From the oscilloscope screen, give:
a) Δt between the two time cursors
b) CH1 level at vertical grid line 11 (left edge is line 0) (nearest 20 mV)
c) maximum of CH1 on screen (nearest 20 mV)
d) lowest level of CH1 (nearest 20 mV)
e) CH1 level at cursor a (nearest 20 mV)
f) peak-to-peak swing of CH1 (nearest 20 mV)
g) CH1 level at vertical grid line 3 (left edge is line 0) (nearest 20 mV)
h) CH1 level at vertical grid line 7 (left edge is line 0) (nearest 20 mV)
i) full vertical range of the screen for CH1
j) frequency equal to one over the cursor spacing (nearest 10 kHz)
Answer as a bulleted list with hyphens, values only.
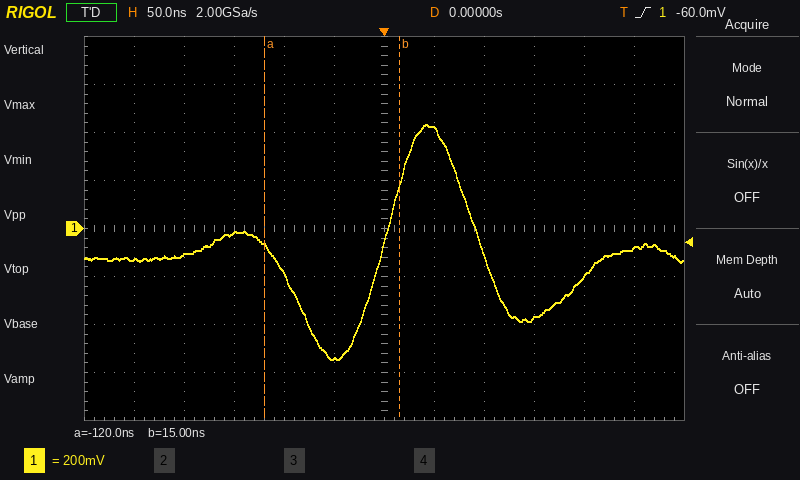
- 135 ns
- -80 mV
- 440 mV
- -540 mV
- -80 mV
- 980 mV
- -20 mV
- 420 mV
- 1.6 V
- 7.41 MHz
